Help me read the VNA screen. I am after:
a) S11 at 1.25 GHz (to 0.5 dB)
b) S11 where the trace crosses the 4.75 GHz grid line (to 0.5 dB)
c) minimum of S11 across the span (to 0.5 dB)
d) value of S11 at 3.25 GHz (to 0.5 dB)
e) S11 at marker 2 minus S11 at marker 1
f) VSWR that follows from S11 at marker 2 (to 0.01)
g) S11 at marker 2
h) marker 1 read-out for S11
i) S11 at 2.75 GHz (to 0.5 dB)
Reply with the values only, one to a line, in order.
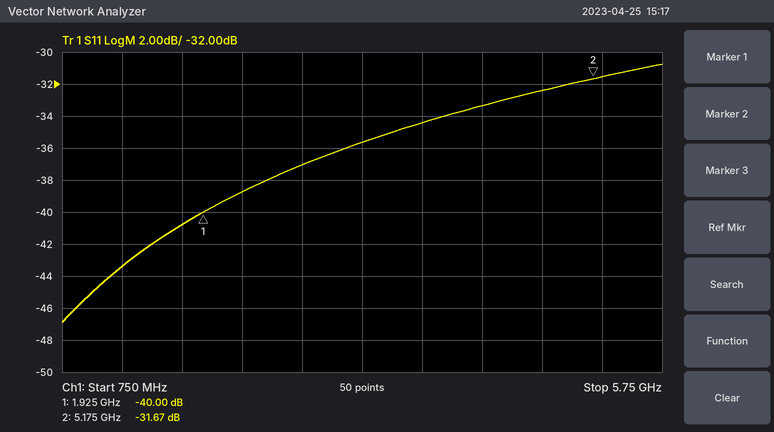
-43.5 dB
-32.5 dB
-47.0 dB
-35.5 dB
8.33 dB
1.05
-31.67 dB
-40.00 dB
-37.0 dB
